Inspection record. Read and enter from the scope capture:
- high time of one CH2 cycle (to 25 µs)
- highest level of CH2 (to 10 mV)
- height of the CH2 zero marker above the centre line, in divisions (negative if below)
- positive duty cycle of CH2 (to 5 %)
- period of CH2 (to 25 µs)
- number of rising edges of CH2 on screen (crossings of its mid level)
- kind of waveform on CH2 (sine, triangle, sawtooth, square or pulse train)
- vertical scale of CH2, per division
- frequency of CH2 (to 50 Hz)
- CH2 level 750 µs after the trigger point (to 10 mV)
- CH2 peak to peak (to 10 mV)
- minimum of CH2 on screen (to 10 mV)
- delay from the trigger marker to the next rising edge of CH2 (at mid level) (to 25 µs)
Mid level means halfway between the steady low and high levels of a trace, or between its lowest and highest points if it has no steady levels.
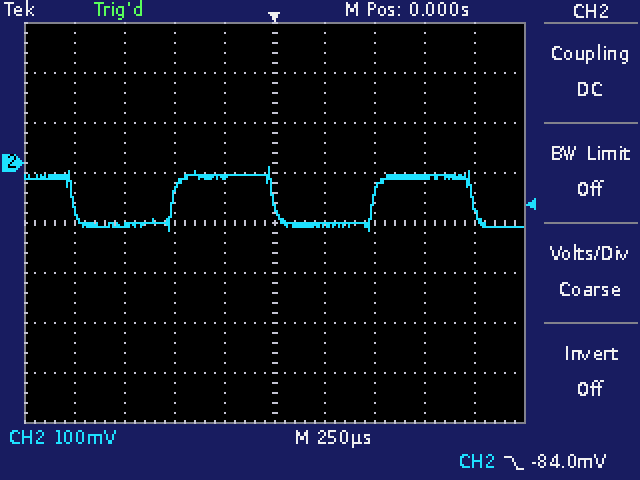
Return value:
500 µs
-10 mV
+1.2 div
50 %
1.000 ms
2
square
100 mV
1.00 kHz
-30 mV
130 mV
-140 mV
500 µs
